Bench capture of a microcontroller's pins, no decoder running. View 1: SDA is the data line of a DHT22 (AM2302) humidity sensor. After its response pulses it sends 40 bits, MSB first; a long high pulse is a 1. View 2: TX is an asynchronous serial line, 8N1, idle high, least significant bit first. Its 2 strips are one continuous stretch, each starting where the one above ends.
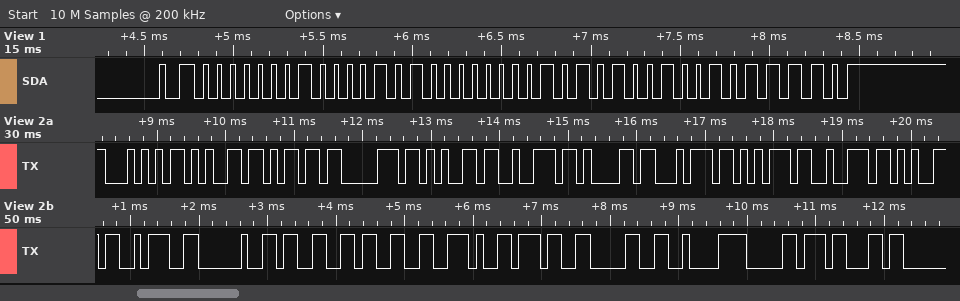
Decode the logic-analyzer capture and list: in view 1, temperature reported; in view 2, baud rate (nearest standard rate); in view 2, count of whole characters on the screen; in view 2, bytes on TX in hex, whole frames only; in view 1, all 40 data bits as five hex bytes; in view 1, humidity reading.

33.8 °C
9600 baud
21
0x54 0x65 0x6D 0x70 0x65 0x72 0x61 0x74 0x75 0x72 0x65 0x3A 0x20 0x33 0x33 0x2E 0x37 0x30 0xC2 0xB0 0x63
01 0A 01 52 5E
26.6 %
